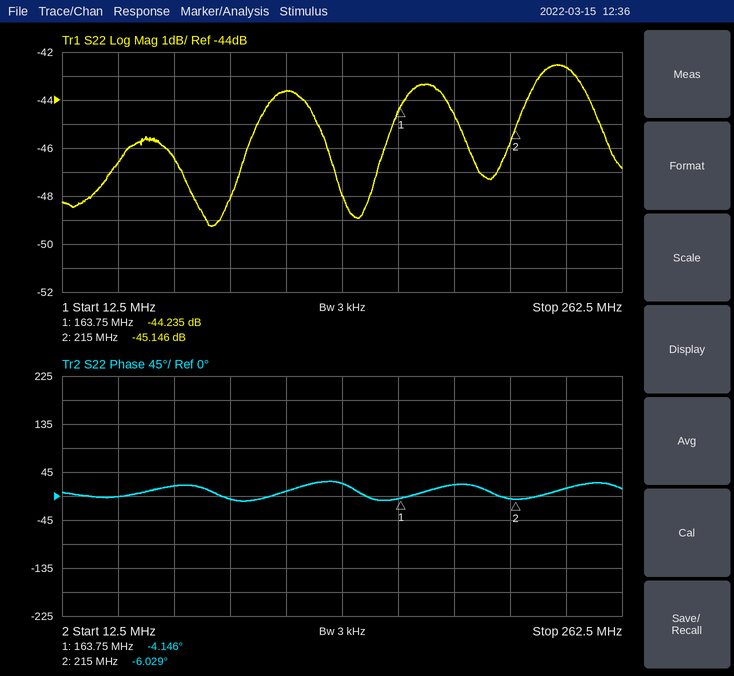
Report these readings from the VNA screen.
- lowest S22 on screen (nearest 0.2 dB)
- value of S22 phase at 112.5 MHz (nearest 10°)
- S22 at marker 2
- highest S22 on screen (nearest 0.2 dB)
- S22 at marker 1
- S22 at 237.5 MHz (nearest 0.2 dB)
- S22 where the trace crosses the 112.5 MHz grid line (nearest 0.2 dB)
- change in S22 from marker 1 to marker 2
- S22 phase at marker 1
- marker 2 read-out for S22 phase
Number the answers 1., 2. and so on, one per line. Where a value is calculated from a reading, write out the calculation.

1. -49.2 dB
2. 10°
3. -45.146 dB
4. -42.6 dB
5. -44.235 dB
6. -42.6 dB
7. -43.6 dB
8. -45.146 − (-44.235) = -0.911 dB
9. -4.146°
10. -6.029°
